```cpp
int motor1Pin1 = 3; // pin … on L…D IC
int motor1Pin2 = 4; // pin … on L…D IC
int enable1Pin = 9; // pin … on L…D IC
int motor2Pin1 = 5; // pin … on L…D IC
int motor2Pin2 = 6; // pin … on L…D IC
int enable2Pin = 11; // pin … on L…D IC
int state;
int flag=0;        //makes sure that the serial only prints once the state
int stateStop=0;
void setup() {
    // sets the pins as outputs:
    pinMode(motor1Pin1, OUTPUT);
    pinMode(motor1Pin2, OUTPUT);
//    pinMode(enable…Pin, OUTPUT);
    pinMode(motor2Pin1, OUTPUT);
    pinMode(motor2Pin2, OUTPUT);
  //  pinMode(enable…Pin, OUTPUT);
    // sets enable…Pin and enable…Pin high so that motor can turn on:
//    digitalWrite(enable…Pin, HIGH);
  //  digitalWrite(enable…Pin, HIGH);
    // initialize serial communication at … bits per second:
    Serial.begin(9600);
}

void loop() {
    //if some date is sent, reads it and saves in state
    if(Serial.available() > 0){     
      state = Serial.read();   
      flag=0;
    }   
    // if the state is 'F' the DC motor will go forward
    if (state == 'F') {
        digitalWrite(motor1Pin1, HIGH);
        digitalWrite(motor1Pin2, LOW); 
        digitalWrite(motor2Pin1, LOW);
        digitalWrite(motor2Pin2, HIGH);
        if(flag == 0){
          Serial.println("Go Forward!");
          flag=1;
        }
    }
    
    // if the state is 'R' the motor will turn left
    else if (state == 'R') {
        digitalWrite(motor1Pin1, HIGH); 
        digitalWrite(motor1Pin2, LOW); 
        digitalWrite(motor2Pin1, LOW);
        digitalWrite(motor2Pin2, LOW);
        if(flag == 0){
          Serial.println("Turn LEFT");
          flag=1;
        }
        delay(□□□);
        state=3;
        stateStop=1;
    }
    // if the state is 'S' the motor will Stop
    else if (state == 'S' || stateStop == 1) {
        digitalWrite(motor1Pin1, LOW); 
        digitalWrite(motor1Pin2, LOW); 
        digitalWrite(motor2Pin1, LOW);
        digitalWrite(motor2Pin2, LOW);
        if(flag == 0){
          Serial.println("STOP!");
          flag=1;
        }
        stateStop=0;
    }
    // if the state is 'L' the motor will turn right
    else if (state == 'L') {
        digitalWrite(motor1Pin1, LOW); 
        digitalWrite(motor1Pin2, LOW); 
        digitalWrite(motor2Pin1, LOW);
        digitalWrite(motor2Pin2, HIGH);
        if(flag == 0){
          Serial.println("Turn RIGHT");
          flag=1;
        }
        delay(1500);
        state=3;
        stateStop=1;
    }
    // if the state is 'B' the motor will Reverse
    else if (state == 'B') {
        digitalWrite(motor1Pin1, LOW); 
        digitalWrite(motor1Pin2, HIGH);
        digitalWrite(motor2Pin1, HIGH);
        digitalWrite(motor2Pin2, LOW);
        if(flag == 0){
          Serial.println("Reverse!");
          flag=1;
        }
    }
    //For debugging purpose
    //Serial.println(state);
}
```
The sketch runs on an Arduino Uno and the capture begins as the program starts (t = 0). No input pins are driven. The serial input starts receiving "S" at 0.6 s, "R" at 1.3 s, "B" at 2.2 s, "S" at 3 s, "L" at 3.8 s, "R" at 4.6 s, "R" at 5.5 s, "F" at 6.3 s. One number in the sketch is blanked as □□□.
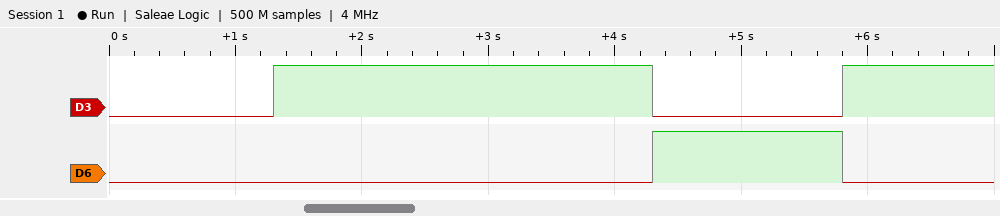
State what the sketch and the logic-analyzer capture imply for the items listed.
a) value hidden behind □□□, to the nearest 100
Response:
3000
